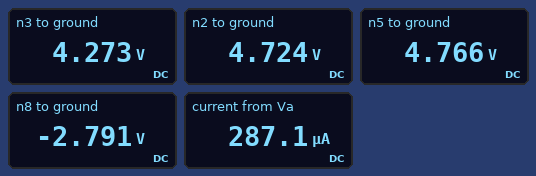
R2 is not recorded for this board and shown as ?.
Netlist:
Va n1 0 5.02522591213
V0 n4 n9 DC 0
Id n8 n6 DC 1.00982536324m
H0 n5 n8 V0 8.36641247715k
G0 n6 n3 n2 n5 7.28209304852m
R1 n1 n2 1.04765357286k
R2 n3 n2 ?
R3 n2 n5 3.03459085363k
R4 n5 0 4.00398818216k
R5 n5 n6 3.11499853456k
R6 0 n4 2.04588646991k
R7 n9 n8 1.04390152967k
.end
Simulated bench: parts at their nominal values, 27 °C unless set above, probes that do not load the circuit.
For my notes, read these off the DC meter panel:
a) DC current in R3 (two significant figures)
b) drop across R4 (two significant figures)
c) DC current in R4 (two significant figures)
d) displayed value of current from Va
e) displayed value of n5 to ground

14 µA
4.8 V
1.2 mA
287.1 µA
4.766 V
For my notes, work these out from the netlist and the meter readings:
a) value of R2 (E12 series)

1.5 kΩ
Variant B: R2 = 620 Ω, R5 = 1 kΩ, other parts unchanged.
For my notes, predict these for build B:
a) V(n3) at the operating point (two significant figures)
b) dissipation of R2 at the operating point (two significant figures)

4.5 V
56 µW
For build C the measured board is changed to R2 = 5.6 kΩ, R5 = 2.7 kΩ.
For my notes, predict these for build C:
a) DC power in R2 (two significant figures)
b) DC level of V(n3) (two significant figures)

510 µW
3.0 V
